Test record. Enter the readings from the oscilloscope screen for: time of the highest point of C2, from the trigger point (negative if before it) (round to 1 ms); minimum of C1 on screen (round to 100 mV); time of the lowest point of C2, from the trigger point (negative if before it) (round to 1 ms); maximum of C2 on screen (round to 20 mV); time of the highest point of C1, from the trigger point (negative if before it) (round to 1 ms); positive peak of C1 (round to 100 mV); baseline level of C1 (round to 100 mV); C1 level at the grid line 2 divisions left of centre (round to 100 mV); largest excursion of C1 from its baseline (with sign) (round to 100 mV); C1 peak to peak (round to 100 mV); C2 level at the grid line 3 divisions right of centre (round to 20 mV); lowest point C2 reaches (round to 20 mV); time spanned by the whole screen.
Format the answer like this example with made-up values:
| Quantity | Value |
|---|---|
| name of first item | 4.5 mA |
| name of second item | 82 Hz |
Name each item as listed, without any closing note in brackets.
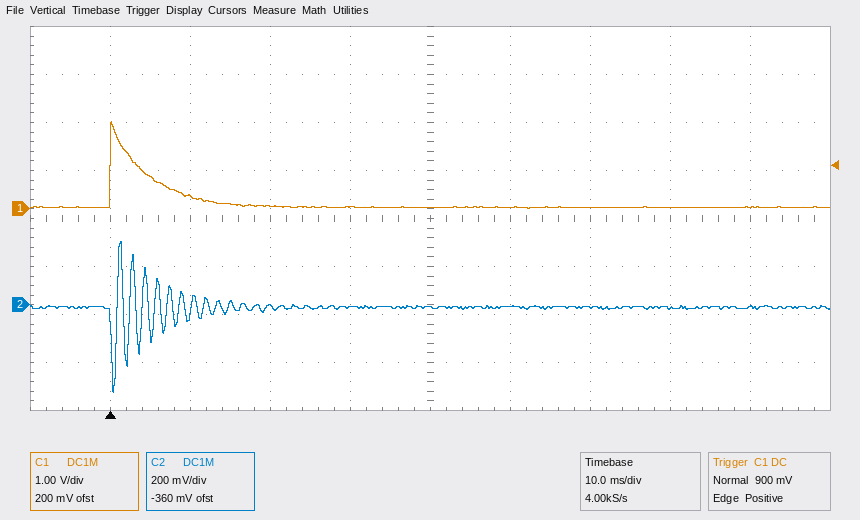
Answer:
| Quantity | Value |
|---|---|
| time of the highest point of C2, from the trigger point (negative if before it) | +1 ms |
| minimum of C1 on screen | 0.0 V |
| time of the lowest point of C2, from the trigger point (negative if before it) | 0 ms |
| maximum of C2 on screen | 260 mV |
| time of the highest point of C1, from the trigger point (negative if before it) | 0 ms |
| positive peak of C1 | 1.8 V |
| baseline level of C1 | 0.0 V |
| C1 level at the grid line 2 divisions left of centre | 100 mV |
| largest excursion of C1 from its baseline (with sign) | +1.8 V |
| C1 peak to peak | 1.8 V |
| C2 level at the grid line 3 divisions right of centre | -20 mV |
| lowest point C2 reaches | -360 mV |
| time spanned by the whole screen | 100 ms |
